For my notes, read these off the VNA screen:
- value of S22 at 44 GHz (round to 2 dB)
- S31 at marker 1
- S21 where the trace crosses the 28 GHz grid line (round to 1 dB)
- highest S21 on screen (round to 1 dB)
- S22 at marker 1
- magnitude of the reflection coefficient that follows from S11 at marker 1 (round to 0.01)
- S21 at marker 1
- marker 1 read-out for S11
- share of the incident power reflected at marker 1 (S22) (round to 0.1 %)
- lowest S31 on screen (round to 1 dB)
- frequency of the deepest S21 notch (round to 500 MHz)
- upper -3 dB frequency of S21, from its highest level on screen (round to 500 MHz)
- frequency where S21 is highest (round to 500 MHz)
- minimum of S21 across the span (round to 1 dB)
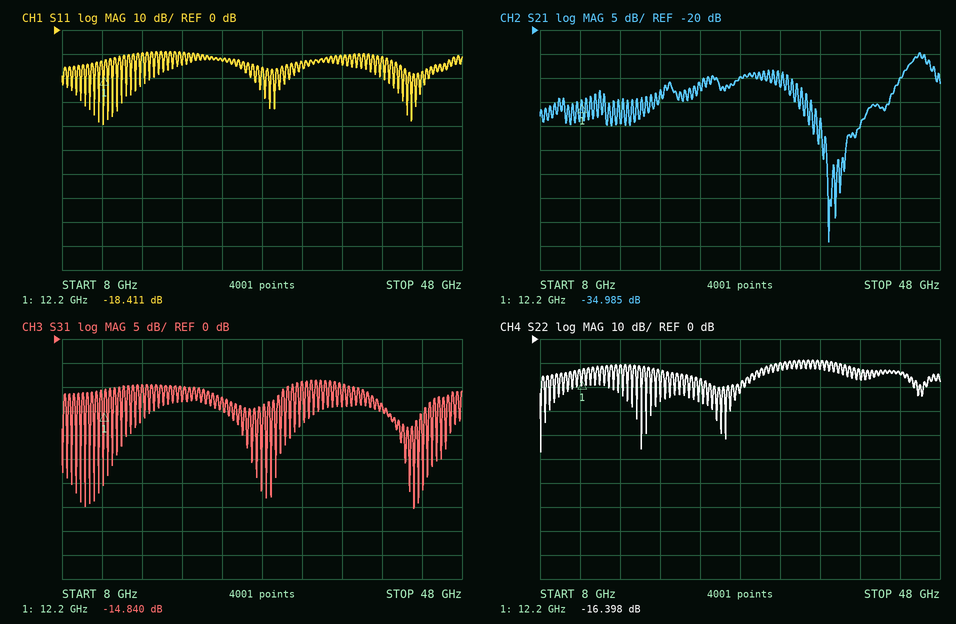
-14 dB
-14.840 dB
-30 dB
-25 dB
-16.398 dB
0.12
-34.985 dB
-18.411 dB
2.3 %
-35 dB
37.0 GHz
47.0 GHz
46.0 GHz
-64 dB
